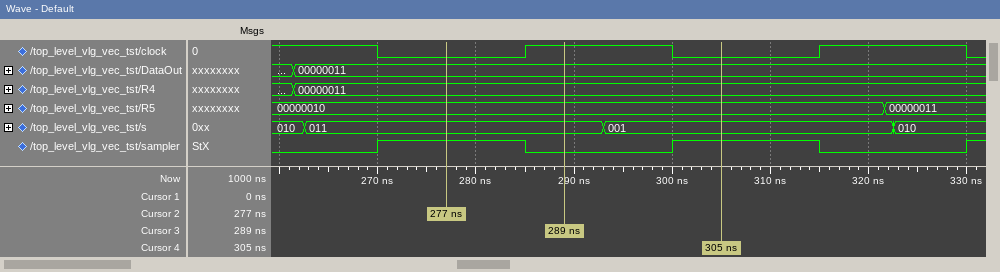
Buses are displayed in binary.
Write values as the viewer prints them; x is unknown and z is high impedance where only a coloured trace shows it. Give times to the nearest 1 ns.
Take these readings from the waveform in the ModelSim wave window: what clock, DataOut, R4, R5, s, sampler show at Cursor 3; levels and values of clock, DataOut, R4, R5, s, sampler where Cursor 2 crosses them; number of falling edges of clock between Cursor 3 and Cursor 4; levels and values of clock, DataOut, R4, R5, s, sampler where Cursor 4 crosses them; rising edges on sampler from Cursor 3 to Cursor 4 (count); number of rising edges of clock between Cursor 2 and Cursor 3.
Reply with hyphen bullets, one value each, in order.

- clock=1, DataOut=00000011, R4=00000011, R5=00000010, s=011, sampler=0
- clock=0, DataOut=00000011, R4=00000011, R5=00000010, s=011, sampler=1
- 1
- clock=0, DataOut=00000011, R4=00000011, R5=00000010, s=001, sampler=1
- 1
- 1
